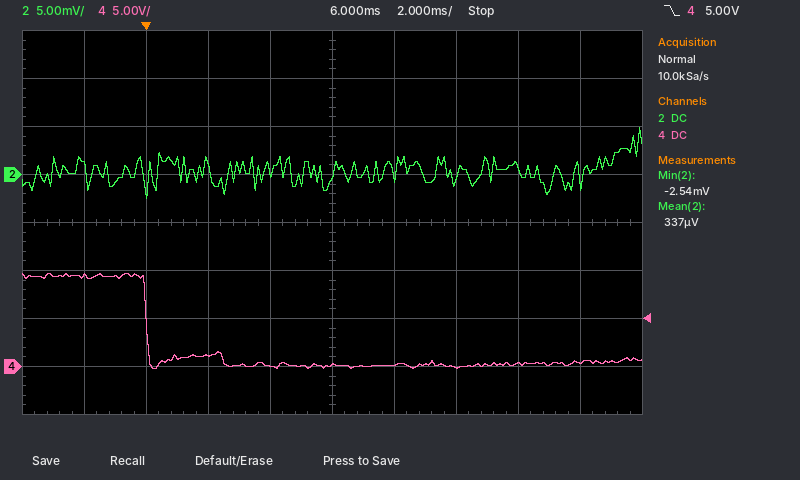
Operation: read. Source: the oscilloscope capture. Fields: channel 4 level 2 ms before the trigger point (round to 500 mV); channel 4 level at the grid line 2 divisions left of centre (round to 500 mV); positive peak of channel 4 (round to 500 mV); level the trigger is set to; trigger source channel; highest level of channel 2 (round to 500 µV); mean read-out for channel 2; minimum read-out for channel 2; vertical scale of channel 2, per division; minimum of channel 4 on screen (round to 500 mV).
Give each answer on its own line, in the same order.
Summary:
9.5 V
1.0 V
9.5 V
5.00 V
channel 4
5.0 mV
337 µV
-2.54 mV
5 mV
0.0 V
